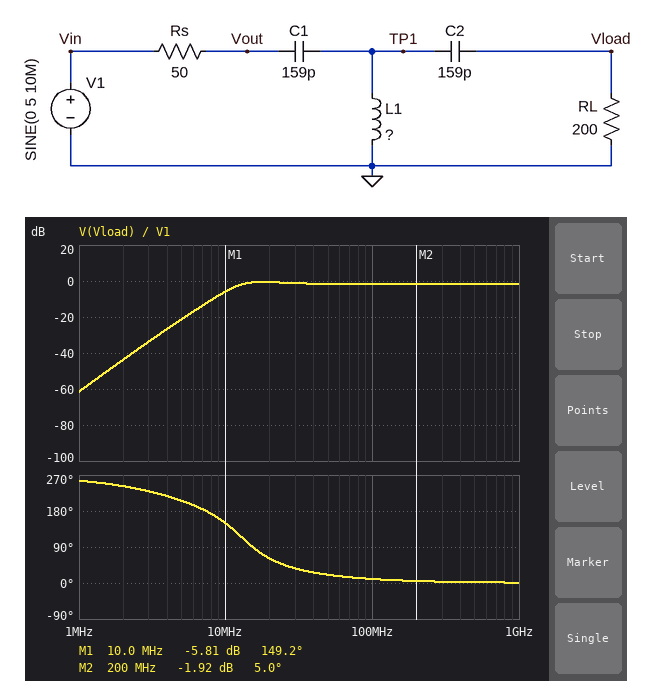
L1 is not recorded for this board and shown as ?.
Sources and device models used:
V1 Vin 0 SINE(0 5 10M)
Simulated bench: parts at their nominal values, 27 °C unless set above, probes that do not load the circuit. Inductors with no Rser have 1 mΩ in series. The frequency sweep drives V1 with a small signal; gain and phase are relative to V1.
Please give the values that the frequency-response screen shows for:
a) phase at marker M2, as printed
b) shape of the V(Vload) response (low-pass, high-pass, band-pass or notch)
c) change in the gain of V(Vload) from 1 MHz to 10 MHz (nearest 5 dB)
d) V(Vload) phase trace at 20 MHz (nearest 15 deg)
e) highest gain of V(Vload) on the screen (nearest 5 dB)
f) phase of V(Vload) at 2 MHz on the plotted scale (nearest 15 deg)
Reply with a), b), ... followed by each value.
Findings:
a) 5.0 deg
b) high-pass
c) 55 dB
d) 60 deg
e) 0 dB
f) 240 deg
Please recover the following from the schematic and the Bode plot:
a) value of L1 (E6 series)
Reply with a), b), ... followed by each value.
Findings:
a) 680 nH
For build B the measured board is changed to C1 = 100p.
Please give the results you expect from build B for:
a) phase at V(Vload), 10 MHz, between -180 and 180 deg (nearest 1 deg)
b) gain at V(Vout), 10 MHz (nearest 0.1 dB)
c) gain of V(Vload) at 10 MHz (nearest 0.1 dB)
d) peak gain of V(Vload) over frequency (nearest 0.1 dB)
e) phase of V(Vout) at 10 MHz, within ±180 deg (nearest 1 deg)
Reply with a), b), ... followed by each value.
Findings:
a) 169 deg
b) -1.0 dB
c) -9.9 dB
d) -0.1 dB
e) -23 deg
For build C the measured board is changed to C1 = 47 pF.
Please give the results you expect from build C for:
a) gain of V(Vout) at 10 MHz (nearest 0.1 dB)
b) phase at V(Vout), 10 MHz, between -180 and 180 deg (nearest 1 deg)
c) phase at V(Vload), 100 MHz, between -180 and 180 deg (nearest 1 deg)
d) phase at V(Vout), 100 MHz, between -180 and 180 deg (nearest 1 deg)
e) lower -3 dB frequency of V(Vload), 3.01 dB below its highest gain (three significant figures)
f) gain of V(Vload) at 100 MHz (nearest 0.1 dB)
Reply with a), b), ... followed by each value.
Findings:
a) -0.2 dB
b) -10 deg
c) 16 deg
d) 3 deg
e) 20.3 MHz
f) -1.7 dB
